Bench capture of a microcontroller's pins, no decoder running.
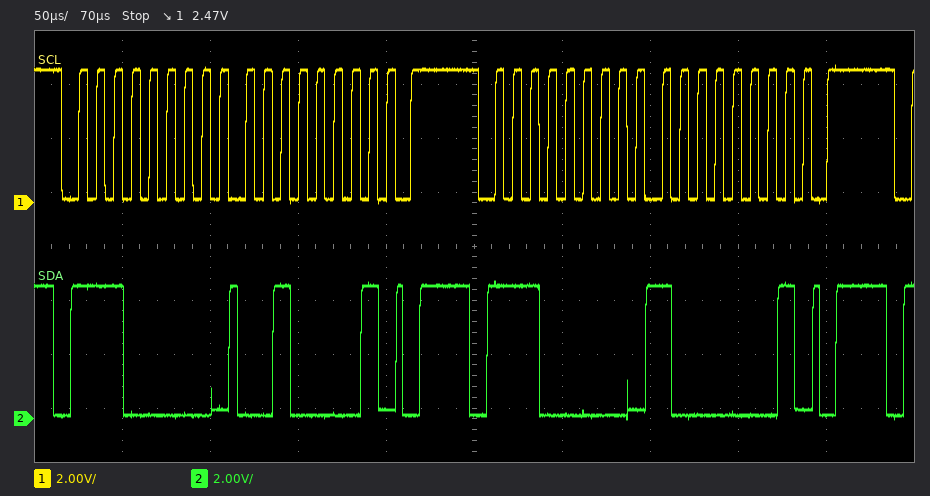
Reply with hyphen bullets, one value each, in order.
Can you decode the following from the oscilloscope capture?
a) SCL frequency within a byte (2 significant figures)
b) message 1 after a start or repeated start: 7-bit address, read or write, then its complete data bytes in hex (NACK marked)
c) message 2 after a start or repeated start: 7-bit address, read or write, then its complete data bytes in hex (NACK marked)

- 100 kHz
- 0x70 write: 21
- 0x70 write: 81
